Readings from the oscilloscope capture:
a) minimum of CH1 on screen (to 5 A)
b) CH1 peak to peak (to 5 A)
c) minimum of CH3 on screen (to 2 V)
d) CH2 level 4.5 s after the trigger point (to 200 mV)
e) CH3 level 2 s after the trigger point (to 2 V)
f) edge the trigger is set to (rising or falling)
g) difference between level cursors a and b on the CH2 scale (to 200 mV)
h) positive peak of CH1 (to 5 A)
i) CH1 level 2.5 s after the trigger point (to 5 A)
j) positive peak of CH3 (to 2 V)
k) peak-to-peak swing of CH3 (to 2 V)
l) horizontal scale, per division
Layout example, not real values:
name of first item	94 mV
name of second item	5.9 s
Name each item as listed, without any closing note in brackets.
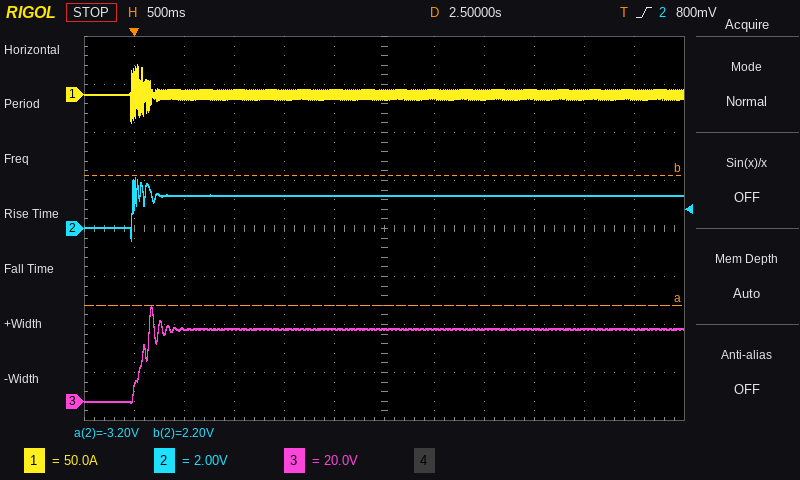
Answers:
minimum of CH1 on screen	-30 A
CH1 peak to peak	60 A
minimum of CH3 on screen	0 V
CH2 level 4.5 s after the trigger point	1.4 V
CH3 level 2 s after the trigger point	30 V
edge the trigger is set to	rising
difference between level cursors a and b on the CH2 scale	5.4 V
positive peak of CH1	30 A
CH1 level 2.5 s after the trigger point	0 A
positive peak of CH3	40 V
peak-to-peak swing of CH3	40 V
horizontal scale, per division	500 ms
